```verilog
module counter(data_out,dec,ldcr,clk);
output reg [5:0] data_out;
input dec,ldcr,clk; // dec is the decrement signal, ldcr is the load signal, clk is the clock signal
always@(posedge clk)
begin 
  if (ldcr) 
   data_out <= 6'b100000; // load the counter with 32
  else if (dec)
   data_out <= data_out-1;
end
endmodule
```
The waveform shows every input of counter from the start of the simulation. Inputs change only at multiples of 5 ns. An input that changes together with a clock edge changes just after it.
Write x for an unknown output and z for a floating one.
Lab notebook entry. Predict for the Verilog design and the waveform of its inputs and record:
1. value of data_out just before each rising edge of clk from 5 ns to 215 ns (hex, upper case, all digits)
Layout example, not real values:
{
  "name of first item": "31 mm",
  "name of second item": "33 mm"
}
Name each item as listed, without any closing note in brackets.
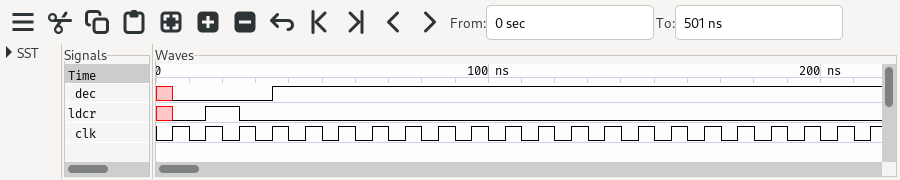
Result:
{
  "value of data_out just before each rising edge of clk from 5 ns to 215 ns": "x, x, x, 20, 20, 1F, 1E, 1D, 1C, 1B, 1A, 19, 18, 17, 16, 15, 14, 13, 12, 11, 10, 0F"
}
